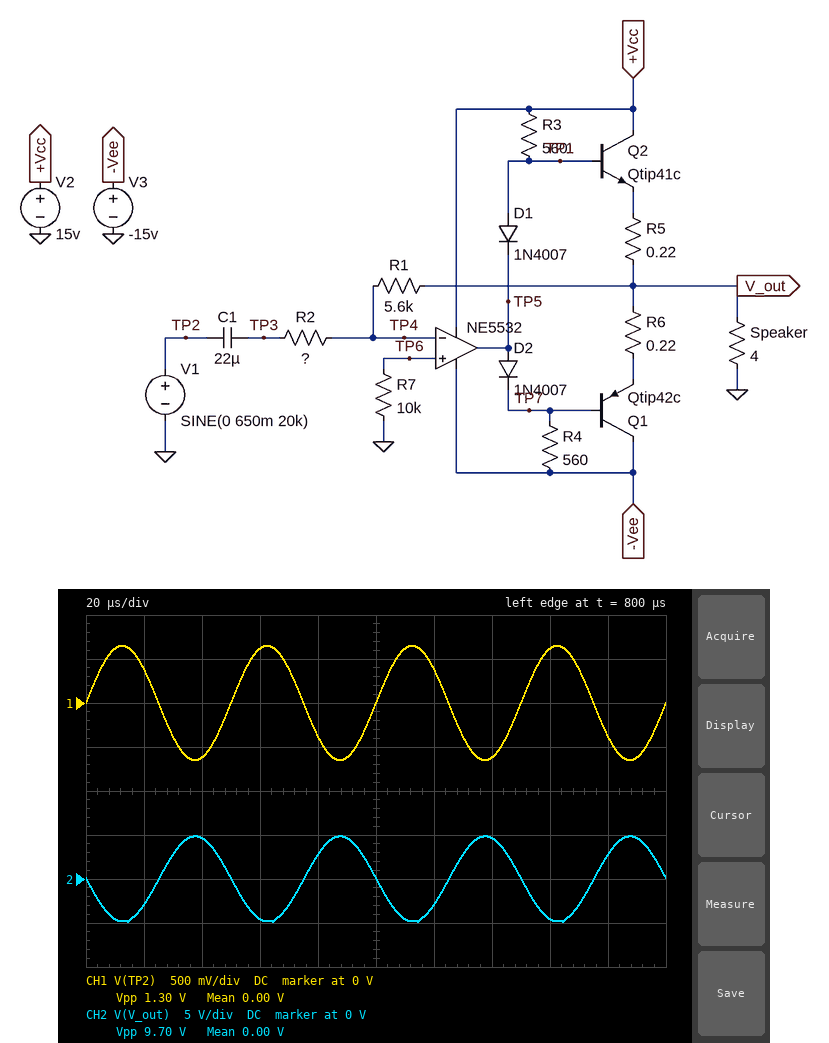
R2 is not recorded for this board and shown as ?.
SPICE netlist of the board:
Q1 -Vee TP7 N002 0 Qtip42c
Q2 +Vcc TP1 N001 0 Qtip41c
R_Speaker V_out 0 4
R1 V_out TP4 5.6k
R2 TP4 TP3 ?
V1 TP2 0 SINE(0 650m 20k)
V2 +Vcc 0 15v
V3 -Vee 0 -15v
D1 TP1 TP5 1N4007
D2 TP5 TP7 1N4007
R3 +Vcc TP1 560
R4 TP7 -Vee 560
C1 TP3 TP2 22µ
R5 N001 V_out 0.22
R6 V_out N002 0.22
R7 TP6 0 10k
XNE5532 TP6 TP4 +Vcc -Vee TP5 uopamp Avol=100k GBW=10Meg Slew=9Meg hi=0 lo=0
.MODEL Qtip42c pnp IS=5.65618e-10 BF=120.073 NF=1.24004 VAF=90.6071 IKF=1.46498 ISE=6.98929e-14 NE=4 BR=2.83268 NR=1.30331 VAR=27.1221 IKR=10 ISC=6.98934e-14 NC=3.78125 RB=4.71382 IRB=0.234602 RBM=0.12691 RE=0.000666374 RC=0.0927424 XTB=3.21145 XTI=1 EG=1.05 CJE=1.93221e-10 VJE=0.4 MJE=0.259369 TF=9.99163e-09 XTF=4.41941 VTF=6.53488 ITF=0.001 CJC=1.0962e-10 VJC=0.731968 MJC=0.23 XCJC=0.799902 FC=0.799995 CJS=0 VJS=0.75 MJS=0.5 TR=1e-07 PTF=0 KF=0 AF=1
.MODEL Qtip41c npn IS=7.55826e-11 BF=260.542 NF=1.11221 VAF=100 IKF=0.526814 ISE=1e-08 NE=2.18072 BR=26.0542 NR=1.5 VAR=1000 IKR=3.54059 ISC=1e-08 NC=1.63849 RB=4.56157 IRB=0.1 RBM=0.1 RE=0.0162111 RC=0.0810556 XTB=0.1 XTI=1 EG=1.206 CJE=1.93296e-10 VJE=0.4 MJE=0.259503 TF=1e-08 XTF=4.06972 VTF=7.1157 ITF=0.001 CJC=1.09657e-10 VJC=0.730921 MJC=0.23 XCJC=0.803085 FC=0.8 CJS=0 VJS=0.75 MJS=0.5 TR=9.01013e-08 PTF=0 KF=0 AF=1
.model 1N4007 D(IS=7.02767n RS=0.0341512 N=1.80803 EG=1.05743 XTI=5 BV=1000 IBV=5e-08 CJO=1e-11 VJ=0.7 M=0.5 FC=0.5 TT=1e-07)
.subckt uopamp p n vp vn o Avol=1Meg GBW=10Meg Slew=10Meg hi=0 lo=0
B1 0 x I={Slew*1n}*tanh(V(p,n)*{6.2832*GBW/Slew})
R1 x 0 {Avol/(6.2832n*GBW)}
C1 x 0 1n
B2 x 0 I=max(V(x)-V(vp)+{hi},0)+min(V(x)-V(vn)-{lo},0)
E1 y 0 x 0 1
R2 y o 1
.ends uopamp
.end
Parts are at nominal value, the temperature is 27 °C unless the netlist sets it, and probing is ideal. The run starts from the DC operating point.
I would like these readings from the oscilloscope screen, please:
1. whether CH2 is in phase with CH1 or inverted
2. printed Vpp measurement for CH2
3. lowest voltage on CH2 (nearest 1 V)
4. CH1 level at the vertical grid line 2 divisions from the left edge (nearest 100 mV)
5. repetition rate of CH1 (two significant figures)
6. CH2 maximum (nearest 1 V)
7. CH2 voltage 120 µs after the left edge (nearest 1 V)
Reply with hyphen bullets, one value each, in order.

- inverted
- 9.70 V
- -5 V
- -600 mV
- 20 kHz
- 5 V
- -3 V
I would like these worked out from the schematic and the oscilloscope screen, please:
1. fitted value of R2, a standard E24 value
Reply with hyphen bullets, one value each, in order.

- 750 Ω
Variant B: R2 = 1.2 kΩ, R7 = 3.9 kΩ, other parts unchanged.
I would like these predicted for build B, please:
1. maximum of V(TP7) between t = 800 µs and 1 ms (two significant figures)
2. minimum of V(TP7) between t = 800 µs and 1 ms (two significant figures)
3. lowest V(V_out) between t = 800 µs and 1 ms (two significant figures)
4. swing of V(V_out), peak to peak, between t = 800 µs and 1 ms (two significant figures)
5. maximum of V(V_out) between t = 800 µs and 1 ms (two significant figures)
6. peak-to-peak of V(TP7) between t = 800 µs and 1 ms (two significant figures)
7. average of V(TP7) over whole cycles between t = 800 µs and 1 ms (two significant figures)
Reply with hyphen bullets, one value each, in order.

- 2.5 V
- -3.9 V
- -3.0 V
- 6.1 V
- 3.0 V
- 6.5 V
- -700 mV
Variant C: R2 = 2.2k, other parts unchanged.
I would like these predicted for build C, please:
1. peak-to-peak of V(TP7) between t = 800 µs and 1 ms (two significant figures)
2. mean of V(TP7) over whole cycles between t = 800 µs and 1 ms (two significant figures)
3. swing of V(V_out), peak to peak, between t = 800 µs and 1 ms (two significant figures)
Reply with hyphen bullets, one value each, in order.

- 3.5 V
- -700 mV
- 3.3 V
